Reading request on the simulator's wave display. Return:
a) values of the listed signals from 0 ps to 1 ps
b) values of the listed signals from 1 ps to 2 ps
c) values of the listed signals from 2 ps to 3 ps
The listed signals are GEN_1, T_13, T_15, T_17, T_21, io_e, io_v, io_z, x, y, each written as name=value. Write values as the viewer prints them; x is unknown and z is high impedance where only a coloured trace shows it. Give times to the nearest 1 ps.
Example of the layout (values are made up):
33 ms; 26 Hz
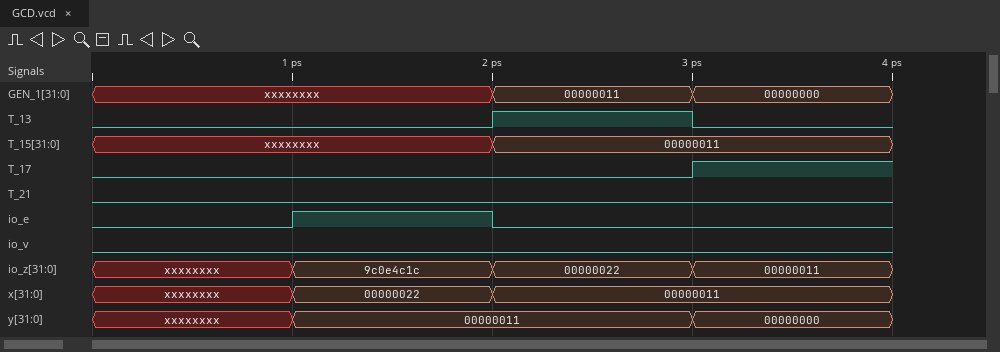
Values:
GEN_1=xxxxxxxx, T_13=0, T_15=xxxxxxxx, T_17=0, T_21=0, io_e=0, io_v=0, io_z=xxxxxxxx, x=xxxxxxxx, y=xxxxxxxx; GEN_1=xxxxxxxx, T_13=0, T_15=xxxxxxxx, T_17=0, T_21=0, io_e=1, io_v=0, io_z=9c0e4c1c, x=00000022, y=00000011; GEN_1=00000011, T_13=1, T_15=00000011, T_17=0, T_21=0, io_e=0, io_v=0, io_z=00000022, x=00000011, y=00000011
